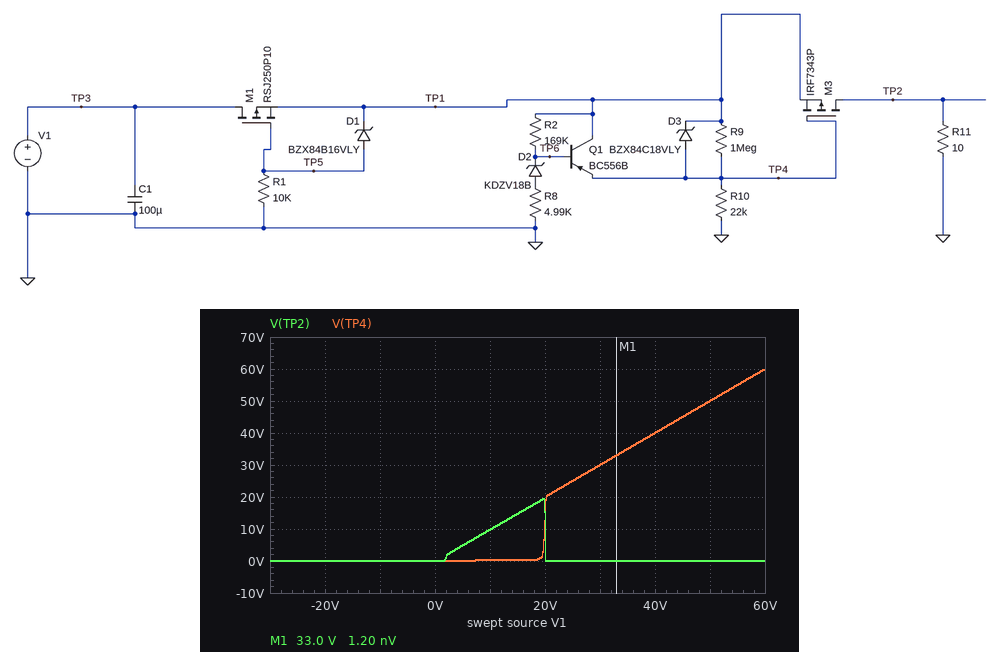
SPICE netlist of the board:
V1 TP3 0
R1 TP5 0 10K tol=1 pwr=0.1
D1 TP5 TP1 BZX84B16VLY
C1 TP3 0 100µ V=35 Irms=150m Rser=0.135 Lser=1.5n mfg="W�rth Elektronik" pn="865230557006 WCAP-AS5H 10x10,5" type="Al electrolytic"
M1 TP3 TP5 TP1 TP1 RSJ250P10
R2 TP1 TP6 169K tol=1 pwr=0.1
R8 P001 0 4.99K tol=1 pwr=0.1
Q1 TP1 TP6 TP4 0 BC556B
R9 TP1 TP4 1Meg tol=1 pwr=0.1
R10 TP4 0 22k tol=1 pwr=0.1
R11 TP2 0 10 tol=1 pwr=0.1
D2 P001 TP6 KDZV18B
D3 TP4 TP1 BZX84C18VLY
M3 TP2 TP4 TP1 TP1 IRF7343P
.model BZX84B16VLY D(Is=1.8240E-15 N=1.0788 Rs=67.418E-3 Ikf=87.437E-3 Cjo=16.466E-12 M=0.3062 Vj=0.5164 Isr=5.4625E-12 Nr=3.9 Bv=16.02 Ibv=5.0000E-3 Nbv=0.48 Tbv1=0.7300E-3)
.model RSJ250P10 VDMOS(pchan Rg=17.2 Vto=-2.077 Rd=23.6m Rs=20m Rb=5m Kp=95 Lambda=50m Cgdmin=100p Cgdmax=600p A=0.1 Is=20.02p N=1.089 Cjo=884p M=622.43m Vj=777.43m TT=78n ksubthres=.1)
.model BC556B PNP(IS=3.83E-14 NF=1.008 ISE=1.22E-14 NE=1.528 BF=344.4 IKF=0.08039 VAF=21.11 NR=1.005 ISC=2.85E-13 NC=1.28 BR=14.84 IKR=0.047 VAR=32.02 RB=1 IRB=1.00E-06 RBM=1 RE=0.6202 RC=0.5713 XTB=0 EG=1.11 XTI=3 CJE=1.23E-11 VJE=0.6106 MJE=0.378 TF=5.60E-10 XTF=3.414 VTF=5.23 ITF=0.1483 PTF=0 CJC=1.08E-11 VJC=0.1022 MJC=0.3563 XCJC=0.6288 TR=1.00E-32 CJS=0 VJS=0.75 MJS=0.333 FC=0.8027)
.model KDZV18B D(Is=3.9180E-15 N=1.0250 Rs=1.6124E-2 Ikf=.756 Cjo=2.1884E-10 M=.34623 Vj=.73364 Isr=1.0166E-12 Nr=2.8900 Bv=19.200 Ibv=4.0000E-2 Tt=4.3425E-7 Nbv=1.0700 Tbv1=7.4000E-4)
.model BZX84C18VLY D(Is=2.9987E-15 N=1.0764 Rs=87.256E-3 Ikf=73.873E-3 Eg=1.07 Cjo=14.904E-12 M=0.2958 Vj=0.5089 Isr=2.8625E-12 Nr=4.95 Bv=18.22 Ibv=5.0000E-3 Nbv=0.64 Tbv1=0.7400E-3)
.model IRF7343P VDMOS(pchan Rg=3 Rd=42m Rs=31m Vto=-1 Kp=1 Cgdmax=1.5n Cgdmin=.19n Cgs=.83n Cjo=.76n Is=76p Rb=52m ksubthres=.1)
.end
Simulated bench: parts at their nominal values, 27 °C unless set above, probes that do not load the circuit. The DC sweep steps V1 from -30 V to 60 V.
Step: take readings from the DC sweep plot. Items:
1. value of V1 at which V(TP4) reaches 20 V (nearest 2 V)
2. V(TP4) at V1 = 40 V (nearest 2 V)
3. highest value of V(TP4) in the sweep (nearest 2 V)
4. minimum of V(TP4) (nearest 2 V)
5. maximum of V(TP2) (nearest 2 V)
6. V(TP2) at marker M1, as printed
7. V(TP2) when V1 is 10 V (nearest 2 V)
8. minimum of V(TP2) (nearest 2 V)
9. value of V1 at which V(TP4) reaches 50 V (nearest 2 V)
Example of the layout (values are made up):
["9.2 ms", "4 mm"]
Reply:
["20 V", "40 V", "60 V", "0 V", "20 V", "1.20 nV", "10 V", "0 V", "50 V"]
